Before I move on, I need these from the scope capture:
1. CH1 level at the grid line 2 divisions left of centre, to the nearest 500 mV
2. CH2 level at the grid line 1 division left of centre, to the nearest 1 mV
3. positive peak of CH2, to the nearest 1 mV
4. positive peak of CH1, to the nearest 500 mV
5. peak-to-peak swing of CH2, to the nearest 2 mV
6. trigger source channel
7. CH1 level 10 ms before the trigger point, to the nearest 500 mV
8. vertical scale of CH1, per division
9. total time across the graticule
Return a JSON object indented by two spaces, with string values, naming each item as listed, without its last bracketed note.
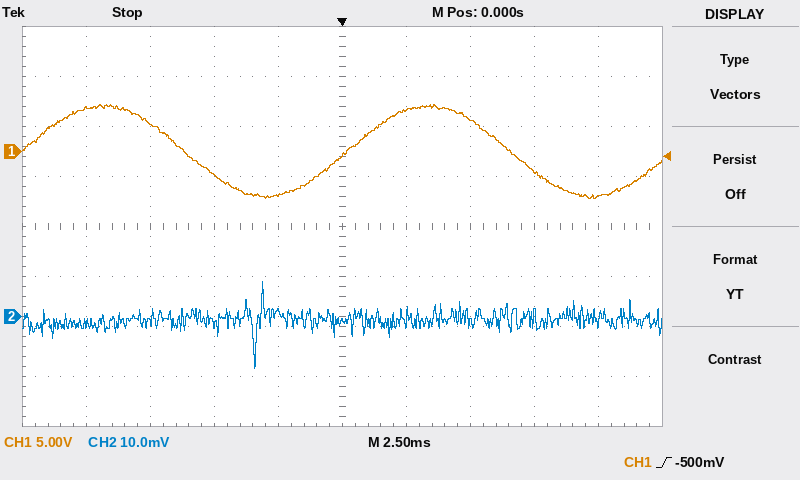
{
  "CH1 level at the grid line 2 divisions left of centre, to the nearest 500 mV": "-2.5 V",
  "CH2 level at the grid line 1 division left of centre, to the nearest 1 mV": "1 mV",
  "positive peak of CH2, to the nearest 1 mV": "7 mV",
  "positive peak of CH1, to the nearest 500 mV": "4.5 V",
  "peak-to-peak swing of CH2, to the nearest 2 mV": "18 mV",
  "trigger source channel": "CH1",
  "CH1 level 10 ms before the trigger point, to the nearest 500 mV": "4.5 V",
  "vertical scale of CH1, per division": "5 V",
  "total time across the graticule": "25 ms"
}
